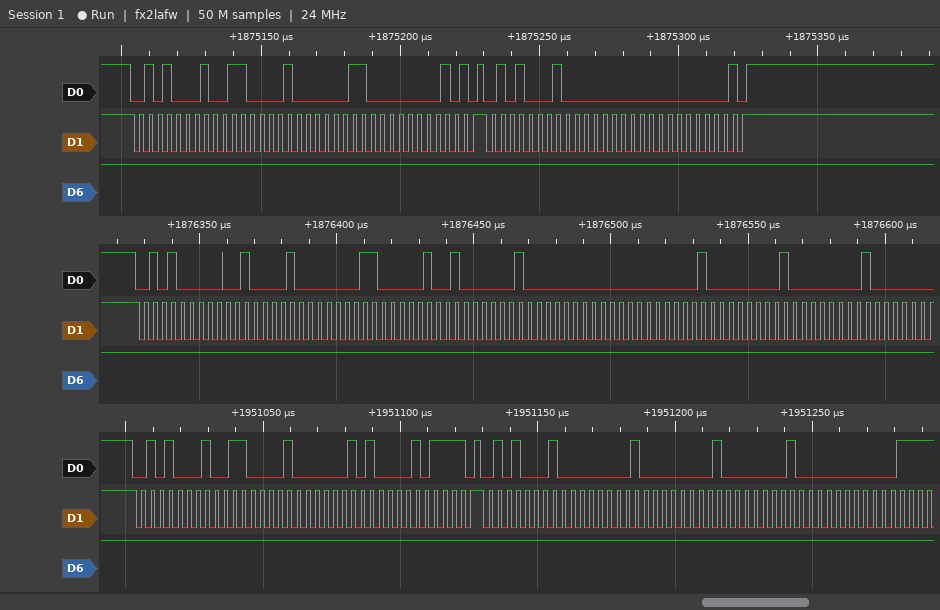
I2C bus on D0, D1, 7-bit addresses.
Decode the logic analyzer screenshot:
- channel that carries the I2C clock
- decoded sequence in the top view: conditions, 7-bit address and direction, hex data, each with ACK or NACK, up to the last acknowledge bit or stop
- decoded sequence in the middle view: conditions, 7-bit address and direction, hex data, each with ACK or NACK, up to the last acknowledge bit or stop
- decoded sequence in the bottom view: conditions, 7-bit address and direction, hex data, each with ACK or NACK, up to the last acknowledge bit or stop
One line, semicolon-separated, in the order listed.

D1; start, address 28 read ACK, 61 ACK, 06 ACK, 02 NACK, stop, start, address 28 read ACK, 00 ACK, 00 NACK, stop; start, address 28 write ACK, 21 ACK, 03 ACK, 09 ACK, 04 ACK, 00 ACK, 01 ACK, 01 ACK, 01 ACK; start, address 28 read ACK, 61 ACK, 05 ACK, 17 NACK, stop, start, address 28 read ACK, 01 ACK, 01 ACK, 02 ACK, 00 ACK
